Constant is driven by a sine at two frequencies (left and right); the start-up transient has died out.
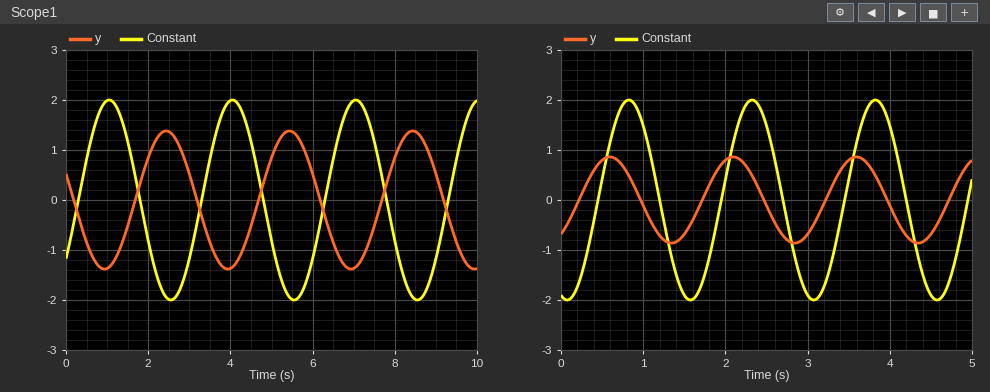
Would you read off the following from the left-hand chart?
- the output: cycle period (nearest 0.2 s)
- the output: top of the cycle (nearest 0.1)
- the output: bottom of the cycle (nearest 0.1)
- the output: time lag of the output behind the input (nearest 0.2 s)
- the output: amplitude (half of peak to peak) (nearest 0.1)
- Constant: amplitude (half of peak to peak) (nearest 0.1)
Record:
3.0 s
1.4
-1.4
1.4 s
1.4
2.0
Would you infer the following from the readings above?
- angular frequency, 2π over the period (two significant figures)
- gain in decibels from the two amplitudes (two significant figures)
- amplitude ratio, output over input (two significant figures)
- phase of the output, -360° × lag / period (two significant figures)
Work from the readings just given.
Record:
2.1 rad/s
-3.1 dB
0.70
-170°
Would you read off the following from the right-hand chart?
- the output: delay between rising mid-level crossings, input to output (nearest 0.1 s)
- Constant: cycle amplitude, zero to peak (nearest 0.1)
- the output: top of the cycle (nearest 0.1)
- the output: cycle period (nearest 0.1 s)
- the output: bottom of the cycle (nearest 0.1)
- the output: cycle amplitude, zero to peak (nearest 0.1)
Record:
1.3 s
2.0
0.9
1.5 s
-0.9
0.9
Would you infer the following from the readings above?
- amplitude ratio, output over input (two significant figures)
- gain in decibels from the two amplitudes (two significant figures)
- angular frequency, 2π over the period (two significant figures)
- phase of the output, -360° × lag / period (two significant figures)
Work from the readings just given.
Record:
0.45
-6.9 dB
4.2 rad/s
-310°
